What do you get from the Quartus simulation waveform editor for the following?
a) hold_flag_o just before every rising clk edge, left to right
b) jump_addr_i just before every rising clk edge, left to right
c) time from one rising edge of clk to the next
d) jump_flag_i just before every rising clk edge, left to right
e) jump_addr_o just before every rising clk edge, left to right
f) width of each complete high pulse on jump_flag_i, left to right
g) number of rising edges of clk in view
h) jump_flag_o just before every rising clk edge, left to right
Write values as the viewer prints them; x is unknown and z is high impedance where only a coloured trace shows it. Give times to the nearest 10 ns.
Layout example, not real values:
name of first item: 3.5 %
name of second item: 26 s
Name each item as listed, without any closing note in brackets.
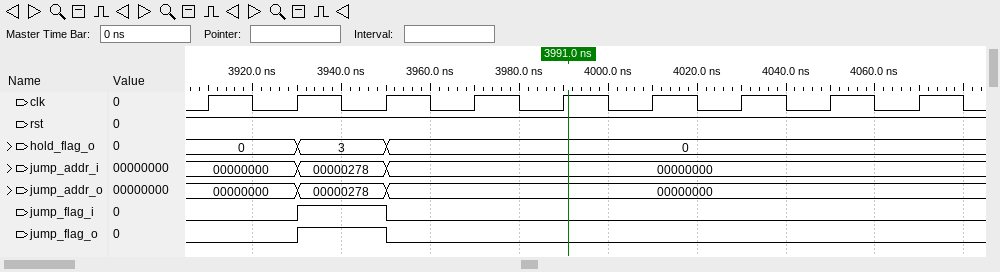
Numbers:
hold_flag_o just before every rising clk edge, left to right: 0, 0, 3, 0, 0, 0, 0, 0, 0
jump_addr_i just before every rising clk edge, left to right: 00000000, 00000000, 00000278, 00000000, 00000000, 00000000, 00000000, 00000000, 00000000
time from one rising edge of clk to the next: 20 ns
jump_flag_i just before every rising clk edge, left to right: 0 0 1 0 0 0 0 0 0
jump_addr_o just before every rising clk edge, left to right: 00000000, 00000000, 00000278, 00000000, 00000000, 00000000, 00000000, 00000000, 00000000
width of each complete high pulse on jump_flag_i, left to right: 20 ns
number of rising edges of clk in view: 9
jump_flag_o just before every rising clk edge, left to right: 0 0 1 0 0 0 0 0 0
